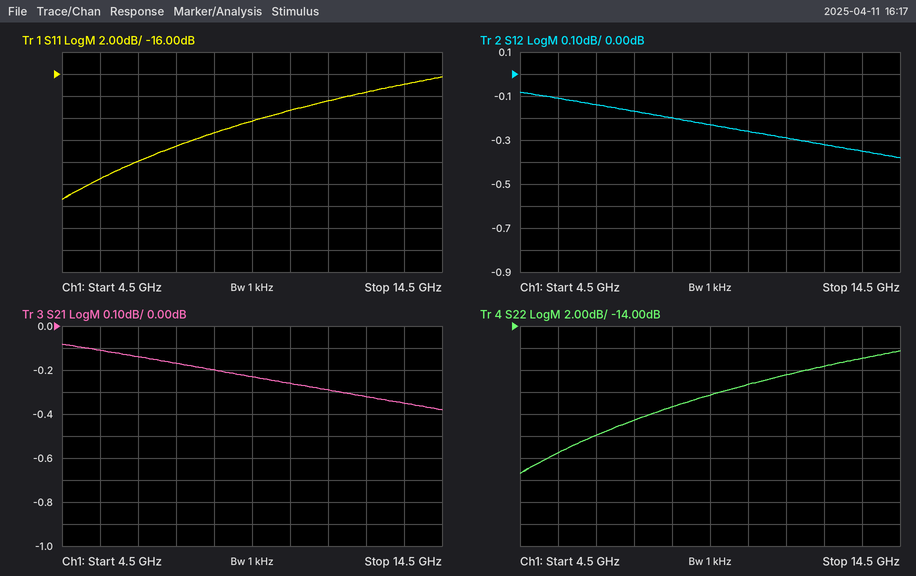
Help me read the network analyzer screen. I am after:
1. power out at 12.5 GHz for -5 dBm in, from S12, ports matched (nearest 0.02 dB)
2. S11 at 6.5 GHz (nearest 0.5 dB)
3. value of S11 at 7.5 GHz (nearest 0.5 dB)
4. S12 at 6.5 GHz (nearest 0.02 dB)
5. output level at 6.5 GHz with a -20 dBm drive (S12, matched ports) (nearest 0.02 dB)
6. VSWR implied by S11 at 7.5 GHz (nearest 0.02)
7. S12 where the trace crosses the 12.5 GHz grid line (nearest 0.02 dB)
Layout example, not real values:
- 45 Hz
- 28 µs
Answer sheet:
- -5.32 dBm
- -24.0 dB
- -22.5 dB
- -0.14 dB
- -20.14 dBm
- 1.16
- -0.32 dB
